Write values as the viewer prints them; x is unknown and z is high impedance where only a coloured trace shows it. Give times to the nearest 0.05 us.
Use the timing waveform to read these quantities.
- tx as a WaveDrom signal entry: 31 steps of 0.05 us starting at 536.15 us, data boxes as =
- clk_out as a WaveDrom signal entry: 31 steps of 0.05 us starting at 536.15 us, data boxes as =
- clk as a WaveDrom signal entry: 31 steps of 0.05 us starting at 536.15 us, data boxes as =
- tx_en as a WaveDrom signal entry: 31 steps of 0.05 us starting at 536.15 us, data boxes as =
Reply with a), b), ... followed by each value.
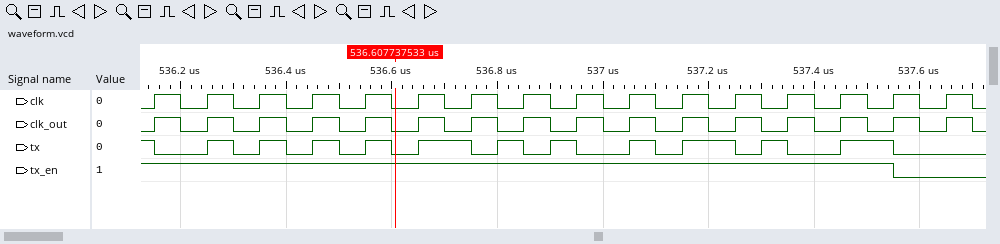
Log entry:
a) {name: 'tx', wave: '0.101010101.01010.101.010.1.0..'}
b) {name: 'clk_out', wave: '1010101010101010101010101010101'}
c) {name: 'clk', wave: '1010101010101010101010101010101'}
d) {name: 'tx_en', wave: '1...........................0..'}
